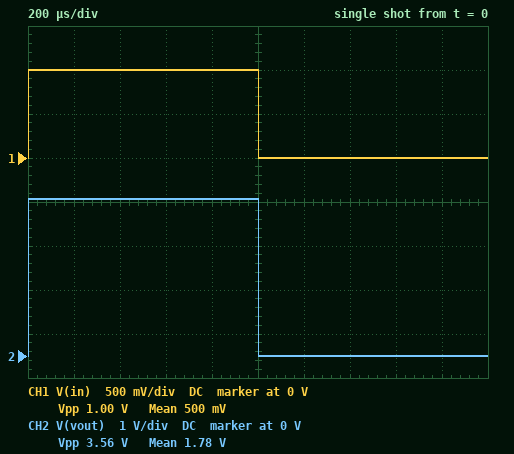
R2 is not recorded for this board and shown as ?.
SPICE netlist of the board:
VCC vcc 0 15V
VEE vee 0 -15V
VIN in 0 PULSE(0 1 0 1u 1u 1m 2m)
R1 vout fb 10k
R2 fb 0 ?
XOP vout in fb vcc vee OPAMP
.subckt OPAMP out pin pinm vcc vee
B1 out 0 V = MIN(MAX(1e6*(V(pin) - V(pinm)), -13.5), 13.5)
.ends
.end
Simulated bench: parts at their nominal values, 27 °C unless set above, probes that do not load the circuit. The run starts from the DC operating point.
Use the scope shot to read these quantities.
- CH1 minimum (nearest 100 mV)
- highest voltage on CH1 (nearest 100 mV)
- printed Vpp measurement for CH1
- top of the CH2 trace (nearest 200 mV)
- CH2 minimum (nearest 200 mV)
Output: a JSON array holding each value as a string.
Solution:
["0 V", "1.0 V", "1.00 V", "3.6 V", "0 V"]
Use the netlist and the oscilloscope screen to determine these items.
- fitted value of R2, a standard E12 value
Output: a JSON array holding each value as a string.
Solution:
["3.9 kΩ"]
